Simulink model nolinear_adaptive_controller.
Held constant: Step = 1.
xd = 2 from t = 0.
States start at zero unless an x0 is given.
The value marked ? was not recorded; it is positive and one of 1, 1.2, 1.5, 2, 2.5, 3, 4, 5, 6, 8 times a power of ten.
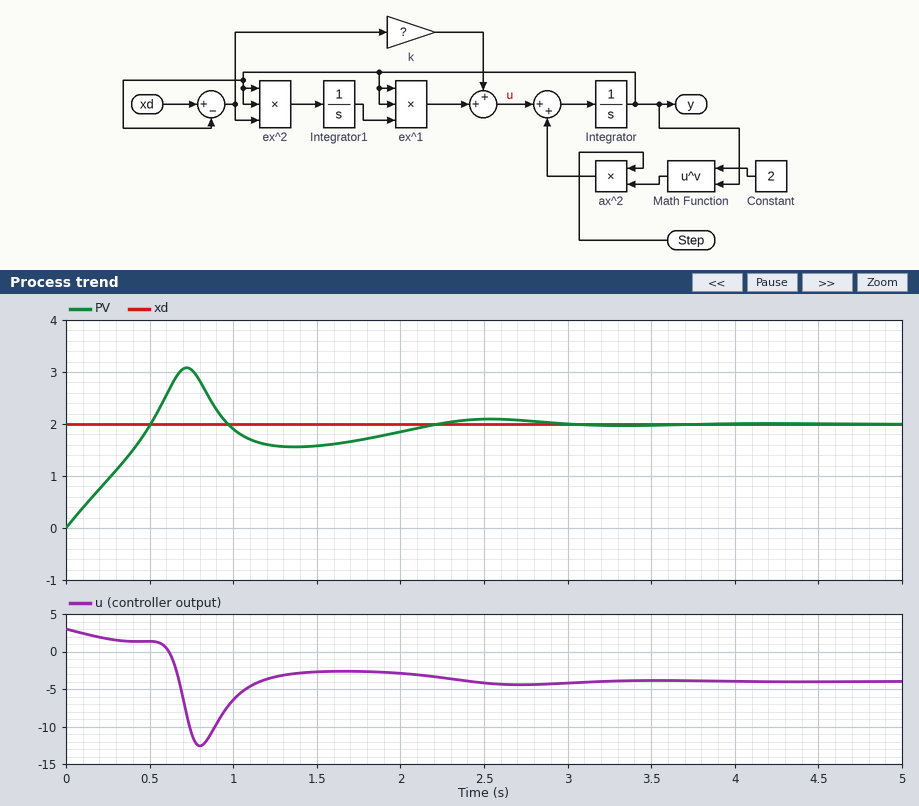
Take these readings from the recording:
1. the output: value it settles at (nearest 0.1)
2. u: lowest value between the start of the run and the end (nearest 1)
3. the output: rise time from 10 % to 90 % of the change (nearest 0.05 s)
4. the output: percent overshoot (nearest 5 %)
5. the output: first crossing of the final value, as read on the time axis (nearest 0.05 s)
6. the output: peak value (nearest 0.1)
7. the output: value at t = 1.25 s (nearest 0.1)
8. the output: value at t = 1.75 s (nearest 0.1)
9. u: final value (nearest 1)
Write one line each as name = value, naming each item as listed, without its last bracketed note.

the output: value it settles at = 2.0
u: lowest value between the start of the run and the end = -13
the output: rise time from 10 % to 90 % of the change = 0.40 s
the output: percent overshoot = 55 %
the output: first crossing of the final value, as read on the time axis = 0.50 s
the output: peak value = 3.1
the output: value at t = 1.25 s = 1.6
the output: value at t = 1.75 s = 1.7
u: final value = -4
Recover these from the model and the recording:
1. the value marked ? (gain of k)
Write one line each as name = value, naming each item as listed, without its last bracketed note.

the value marked ? = 1.5
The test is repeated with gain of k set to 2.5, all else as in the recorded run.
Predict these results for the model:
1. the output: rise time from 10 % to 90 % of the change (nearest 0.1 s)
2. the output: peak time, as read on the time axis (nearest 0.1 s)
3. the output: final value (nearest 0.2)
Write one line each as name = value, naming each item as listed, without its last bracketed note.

the output: rise time from 10 % to 90 % of the change = 0.3 s
the output: peak time, as read on the time axis = 0.6 s
the output: final value = 2.0
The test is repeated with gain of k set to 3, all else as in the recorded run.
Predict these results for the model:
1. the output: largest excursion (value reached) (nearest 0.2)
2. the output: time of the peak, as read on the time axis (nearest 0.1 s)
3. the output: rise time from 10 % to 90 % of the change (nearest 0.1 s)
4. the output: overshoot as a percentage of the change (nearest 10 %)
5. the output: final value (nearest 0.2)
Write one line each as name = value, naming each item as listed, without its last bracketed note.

the output: largest excursion (value reached) = 2.8
the output: time of the peak, as read on the time axis = 0.6 s
the output: rise time from 10 % to 90 % of the change = 0.3 s
the output: overshoot as a percentage of the change = 40 %
the output: final value = 2.0
